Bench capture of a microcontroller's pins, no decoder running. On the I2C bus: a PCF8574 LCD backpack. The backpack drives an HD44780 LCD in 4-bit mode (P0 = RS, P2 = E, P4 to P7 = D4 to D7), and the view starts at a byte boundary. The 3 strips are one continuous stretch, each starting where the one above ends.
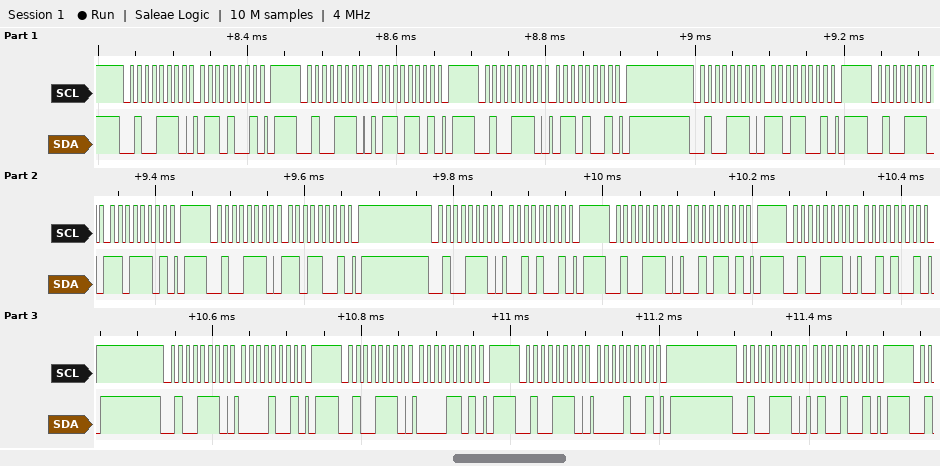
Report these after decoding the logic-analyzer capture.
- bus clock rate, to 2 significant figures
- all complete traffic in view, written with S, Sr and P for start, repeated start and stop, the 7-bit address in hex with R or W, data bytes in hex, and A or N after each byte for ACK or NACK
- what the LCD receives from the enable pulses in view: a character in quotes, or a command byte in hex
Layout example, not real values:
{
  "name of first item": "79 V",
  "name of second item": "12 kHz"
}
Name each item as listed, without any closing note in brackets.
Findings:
{
  "bus clock rate, to 2 significant figures": "100 kHz",
  "all complete traffic in view, written with S, Sr and P for start, repeated start and stop, the 7-bit address in hex with R or W, data bytes in hex, and A or N after each byte for ACK or NACK": "S 27W A 69 A P S 27W A 6D A P S 27W A 69 A P S 27W A D9 A P S 27W A DD A P S 27W A D9 A P S 27W A 29 A P S 27W A 2D A P S 27W A 29 A P S 27W A 09 A P S 27W A 0D A P S 27W A 09 A P S 27W A 49 A P",
  "what the LCD receives from the enable pulses in view: a character in quotes, or a command byte in hex": "'m' ' '"
}
